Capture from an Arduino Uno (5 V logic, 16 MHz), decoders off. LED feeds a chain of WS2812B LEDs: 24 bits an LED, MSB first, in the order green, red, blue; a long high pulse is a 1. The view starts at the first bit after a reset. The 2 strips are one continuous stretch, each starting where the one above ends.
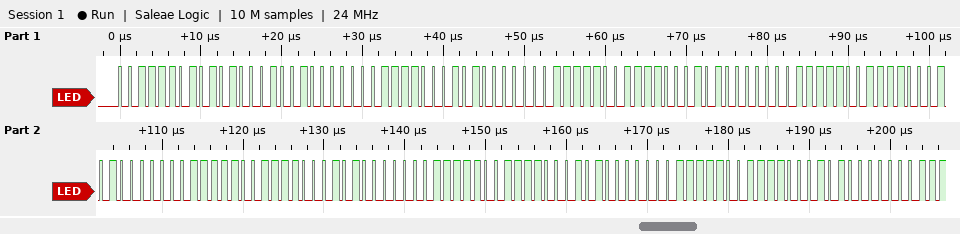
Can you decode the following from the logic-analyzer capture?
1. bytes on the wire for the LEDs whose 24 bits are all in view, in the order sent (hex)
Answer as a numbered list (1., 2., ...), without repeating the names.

1. 3D 51 20 3C 50 1F 3C 50 1F 3C 50 1F 3C 50 1F 3C 50 1F
